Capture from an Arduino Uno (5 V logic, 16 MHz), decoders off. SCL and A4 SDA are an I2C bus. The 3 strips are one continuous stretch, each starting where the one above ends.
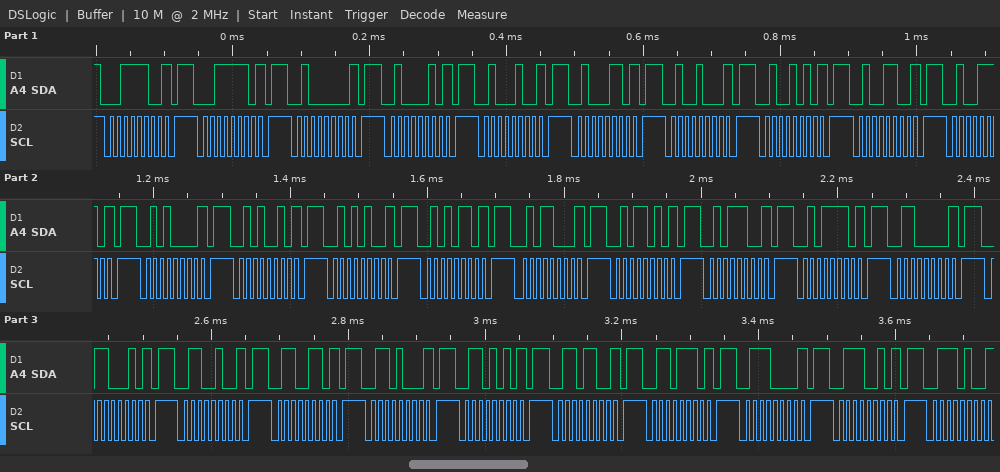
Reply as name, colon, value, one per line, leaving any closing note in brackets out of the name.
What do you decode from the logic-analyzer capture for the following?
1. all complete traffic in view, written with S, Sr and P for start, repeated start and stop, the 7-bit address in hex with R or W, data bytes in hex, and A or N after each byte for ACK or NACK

all complete traffic in view, written with S, Sr and P for start, repeated start and stop, the 7-bit address in hex with R or W, data bytes in hex, and A or N after each byte for ACK or NACK: S 1EW N P S 1FW N P S 20W N P S 21W N P S 22W N P S 23W N P S 24W N P S 25W N P S 26W N P S 27W N P S 28W N P S 29W N P S 2AW N P S 2BW N P S 2CW N P S 2DW N P S 2EW N P S 2FW N P S 30W N P S 31W N P S 32W N P S 33W N P S 34W N P S 35W N P S 36W N P S 37W N P S 38W N P S 39W N P S 3AW N
